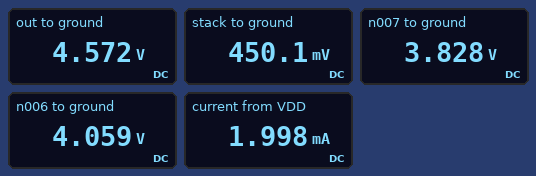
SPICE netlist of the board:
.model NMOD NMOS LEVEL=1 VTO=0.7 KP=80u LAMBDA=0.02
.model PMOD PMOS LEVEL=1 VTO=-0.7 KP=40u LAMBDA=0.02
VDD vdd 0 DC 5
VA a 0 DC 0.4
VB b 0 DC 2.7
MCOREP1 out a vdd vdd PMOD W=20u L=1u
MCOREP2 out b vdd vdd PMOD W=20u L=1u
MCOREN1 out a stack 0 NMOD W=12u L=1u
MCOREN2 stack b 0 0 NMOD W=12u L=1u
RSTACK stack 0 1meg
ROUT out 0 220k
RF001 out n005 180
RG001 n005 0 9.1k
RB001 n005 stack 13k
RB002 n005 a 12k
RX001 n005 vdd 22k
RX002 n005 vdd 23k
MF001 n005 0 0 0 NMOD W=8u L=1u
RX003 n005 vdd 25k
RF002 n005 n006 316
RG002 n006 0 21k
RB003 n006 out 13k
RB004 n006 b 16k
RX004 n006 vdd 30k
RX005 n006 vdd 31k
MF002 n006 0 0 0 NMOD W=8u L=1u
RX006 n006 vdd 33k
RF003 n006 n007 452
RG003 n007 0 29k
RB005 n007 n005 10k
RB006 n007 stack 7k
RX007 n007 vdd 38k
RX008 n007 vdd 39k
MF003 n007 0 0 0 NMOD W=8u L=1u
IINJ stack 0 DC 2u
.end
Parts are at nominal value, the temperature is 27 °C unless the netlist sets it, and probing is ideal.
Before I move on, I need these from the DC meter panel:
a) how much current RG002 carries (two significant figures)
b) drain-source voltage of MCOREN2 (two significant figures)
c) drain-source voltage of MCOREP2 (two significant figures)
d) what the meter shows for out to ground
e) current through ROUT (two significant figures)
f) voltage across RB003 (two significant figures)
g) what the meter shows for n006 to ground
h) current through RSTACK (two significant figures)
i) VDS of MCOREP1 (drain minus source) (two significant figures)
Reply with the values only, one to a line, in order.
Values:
190 µA
450 mV
-430 mV
4.572 V
21 µA
510 mV
4.059 V
450 nA
-430 mV
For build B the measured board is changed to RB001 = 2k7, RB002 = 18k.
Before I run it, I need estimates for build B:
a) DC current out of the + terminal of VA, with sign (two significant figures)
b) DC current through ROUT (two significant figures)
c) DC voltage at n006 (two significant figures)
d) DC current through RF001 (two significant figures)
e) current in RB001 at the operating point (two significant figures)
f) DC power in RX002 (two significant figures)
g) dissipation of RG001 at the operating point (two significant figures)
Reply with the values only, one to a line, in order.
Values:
-200 µA
20 µA
3.9 V
2.2 mA
1.1 mA
40 µW
1.8 mW
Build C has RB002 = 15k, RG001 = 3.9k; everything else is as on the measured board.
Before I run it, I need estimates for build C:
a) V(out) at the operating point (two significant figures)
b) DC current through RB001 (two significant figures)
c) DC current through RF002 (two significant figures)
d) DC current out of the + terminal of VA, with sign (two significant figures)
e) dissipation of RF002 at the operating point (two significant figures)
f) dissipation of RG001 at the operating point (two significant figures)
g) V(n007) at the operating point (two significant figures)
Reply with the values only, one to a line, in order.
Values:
4.5 V
280 µA
590 µA
-250 µA
110 µW
4.3 mW
3.7 V
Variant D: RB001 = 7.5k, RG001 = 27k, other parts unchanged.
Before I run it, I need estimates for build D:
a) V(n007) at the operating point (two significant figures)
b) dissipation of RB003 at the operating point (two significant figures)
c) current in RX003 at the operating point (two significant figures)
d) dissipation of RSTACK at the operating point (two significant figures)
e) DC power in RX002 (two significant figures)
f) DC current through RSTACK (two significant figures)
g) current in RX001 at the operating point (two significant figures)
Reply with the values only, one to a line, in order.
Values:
3.9 V
19 µW
28 µA
340 nW
21 µW
580 nA
31 µA
